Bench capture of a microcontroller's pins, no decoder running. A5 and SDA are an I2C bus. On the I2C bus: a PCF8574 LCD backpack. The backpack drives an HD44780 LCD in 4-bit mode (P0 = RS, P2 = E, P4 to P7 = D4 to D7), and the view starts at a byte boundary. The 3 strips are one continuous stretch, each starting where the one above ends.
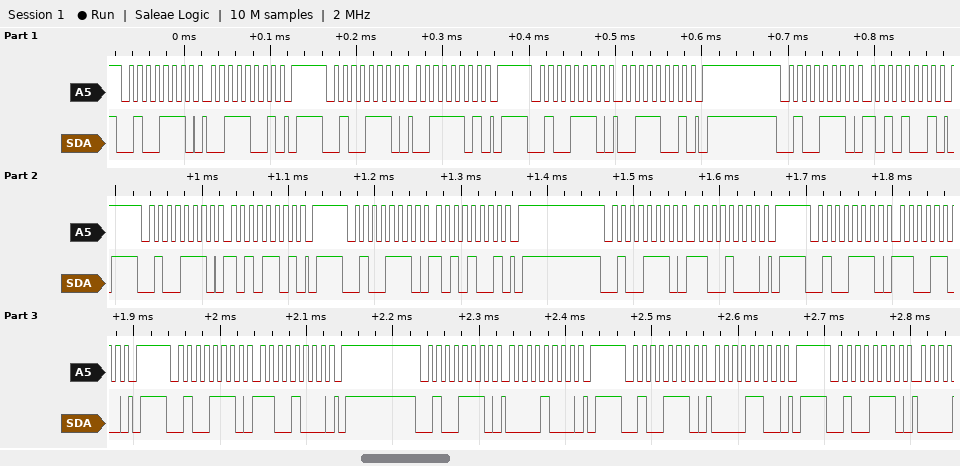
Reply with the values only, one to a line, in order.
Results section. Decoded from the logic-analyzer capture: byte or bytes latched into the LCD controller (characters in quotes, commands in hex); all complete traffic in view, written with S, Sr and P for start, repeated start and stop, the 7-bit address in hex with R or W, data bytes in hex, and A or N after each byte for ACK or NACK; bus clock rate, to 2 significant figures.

':'
S 27W A 39 A P S 27W A 3D A P S 27W A 39 A P S 27W A A9 A P S 27W A AD A P S 27W A A9 A P S 27W A C8 A P S 27W A CC A P S 27W A C8 A P S 27W A 08 A P S 27W A 0C A P S 27W A
100 kHz
